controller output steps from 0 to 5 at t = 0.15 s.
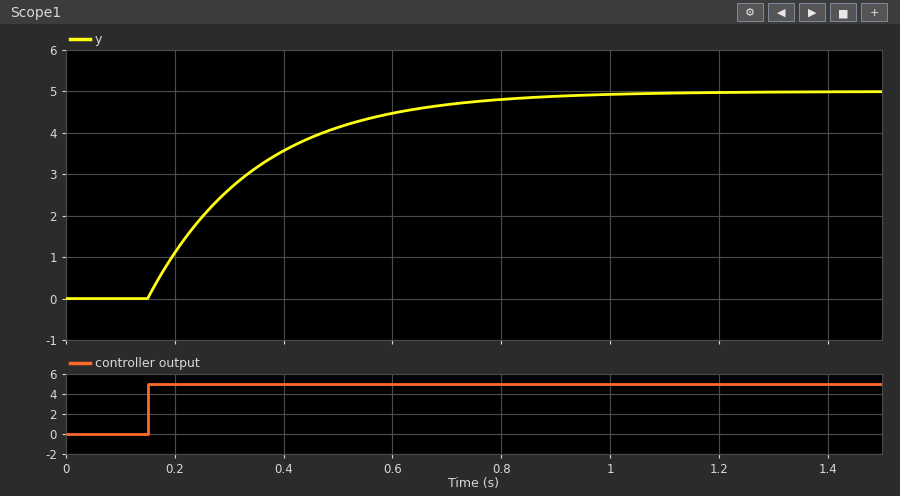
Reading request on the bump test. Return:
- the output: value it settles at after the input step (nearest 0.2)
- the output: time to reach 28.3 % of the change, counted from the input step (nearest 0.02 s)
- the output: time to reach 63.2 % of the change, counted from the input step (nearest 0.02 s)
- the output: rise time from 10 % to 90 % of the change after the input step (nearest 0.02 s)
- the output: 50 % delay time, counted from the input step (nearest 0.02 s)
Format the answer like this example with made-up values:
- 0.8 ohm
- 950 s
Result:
- 5.0
- 0.06 s
- 0.20 s
- 0.44 s
- 0.14 s
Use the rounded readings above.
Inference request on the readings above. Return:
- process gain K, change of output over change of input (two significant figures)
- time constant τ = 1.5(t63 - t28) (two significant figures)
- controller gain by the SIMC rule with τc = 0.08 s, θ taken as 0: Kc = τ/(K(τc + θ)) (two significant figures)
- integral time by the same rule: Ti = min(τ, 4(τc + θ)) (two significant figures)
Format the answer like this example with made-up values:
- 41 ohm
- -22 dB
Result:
- 1.0
- 0.21 s
- 2.6
- 0.21 s
